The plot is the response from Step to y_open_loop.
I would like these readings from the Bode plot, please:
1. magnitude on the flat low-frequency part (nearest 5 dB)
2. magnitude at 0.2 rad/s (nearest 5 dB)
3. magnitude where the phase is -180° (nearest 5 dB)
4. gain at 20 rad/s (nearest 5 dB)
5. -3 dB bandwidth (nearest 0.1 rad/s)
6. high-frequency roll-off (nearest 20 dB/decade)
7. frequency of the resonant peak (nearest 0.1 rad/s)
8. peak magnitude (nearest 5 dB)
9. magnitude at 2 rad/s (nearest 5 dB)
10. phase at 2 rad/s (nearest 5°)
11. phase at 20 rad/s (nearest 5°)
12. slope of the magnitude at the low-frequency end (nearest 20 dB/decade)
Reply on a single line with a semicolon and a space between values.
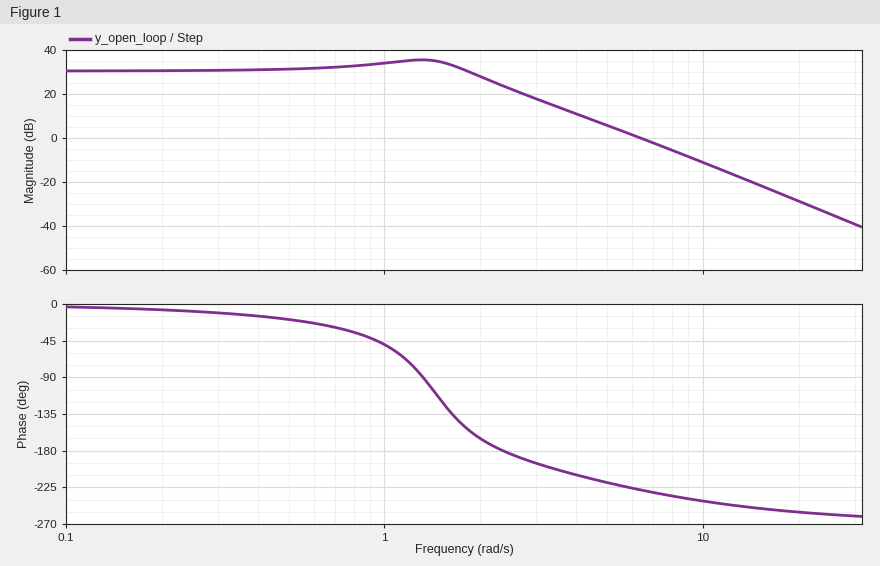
30 dB; 30 dB; 25 dB; -30 dB; 2.0 rad/s; -60 dB/decade; 1.3 rad/s; 35 dB; 30 dB; -165°; -255°; 0 dB/decade
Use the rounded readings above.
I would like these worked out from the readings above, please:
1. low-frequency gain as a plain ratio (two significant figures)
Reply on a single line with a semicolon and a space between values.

32
